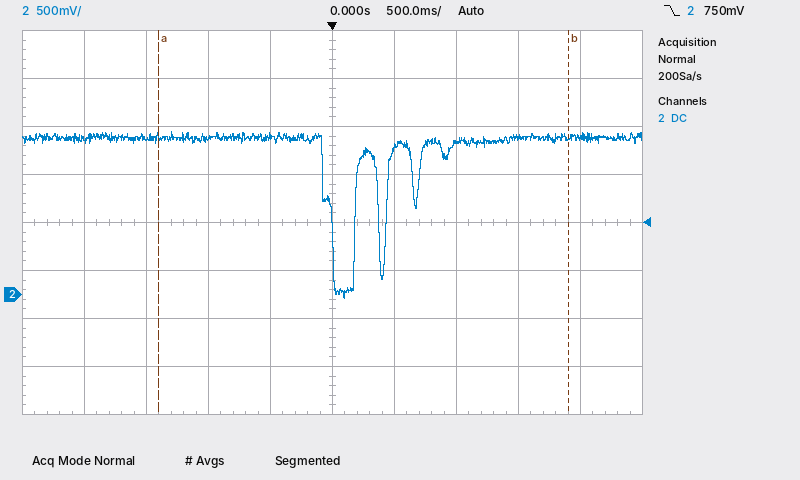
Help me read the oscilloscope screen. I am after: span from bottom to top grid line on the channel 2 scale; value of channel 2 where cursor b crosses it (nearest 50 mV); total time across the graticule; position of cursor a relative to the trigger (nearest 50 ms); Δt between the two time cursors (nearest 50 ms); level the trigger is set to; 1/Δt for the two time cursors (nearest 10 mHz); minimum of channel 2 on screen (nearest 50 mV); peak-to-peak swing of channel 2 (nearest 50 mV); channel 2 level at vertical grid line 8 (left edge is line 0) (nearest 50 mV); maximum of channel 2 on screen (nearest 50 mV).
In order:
4 V
1.65 V
5 s
-1.40 s
3.30 s
750 mV
300 mHz
-50 mV
1.75 V
1.65 V
1.70 V
